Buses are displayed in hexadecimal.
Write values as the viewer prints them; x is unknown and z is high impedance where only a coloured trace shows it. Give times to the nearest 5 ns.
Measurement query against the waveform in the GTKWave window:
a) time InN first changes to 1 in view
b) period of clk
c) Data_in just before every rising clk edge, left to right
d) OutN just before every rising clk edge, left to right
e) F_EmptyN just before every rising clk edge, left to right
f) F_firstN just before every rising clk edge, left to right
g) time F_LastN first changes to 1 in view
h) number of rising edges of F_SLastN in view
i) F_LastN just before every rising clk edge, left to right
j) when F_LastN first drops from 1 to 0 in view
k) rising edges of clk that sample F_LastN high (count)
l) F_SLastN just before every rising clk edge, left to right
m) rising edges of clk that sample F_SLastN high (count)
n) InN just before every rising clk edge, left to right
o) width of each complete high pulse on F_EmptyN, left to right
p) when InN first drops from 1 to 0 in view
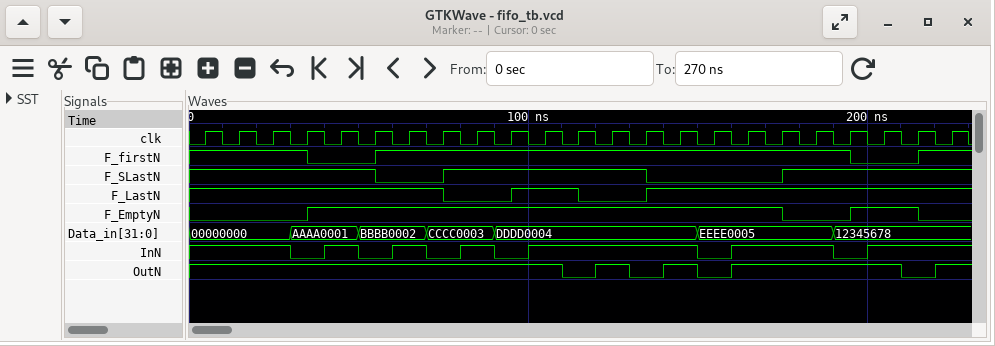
40 ns
10 ns
00000000, 00000000, 00000000, AAAA0001, AAAA0001, BBBB0002, BBBB0002, CCCC0003, CCCC0003, DDDD0004, DDDD0004, DDDD0004, DDDD0004, DDDD0004, DDDD0004, EEEE0005, EEEE0005, EEEE0005, EEEE0005, 12345678, 12345678, 12345678, 12345678
1 1 1 1 1 1 1 1 1 1 1 0 1 0 1 0 1 1 1 1 1 0 1
0 0 0 0 1 1 1 1 1 1 1 1 1 1 1 1 1 1 0 0 1 1 0
1 1 1 1 0 0 1 1 1 1 1 1 1 1 1 1 1 1 1 1 0 0 1
95 ns
2
1 1 1 1 1 1 1 1 0 0 1 1 0 0 1 1 1 1 1 1 1 1 1
75 ns
19
1 1 1 1 1 1 0 0 1 1 1 1 1 1 0 0 0 0 1 1 1 1 1
17
1 1 1 0 1 0 1 0 1 0 1 1 1 1 1 0 1 1 1 0 1 1 1
140 ns, 20 ns
30 ns
